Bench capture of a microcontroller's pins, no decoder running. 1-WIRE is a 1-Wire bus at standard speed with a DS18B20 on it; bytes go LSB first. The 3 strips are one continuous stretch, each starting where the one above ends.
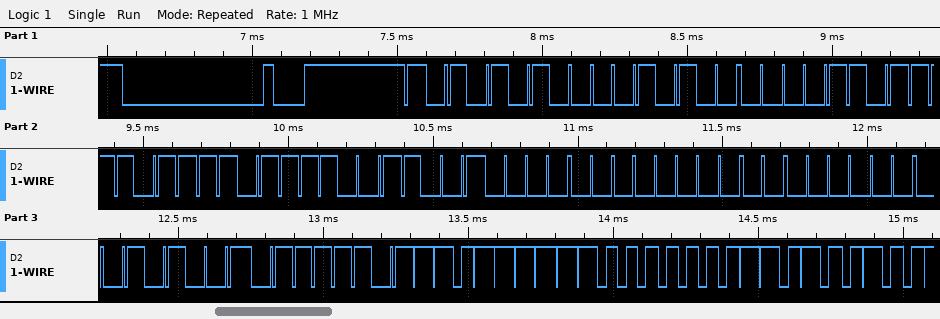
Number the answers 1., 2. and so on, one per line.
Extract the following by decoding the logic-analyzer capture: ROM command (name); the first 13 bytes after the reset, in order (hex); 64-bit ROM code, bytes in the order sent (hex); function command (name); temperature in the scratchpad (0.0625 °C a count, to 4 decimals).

1. Match ROM
2. 55 28 B0 F7 9E 09 00 00 94 BE FB 01 4B
3. 28 B0 F7 9E 09 00 00 94
4. Read Scratchpad
5. 31.6875 °C
